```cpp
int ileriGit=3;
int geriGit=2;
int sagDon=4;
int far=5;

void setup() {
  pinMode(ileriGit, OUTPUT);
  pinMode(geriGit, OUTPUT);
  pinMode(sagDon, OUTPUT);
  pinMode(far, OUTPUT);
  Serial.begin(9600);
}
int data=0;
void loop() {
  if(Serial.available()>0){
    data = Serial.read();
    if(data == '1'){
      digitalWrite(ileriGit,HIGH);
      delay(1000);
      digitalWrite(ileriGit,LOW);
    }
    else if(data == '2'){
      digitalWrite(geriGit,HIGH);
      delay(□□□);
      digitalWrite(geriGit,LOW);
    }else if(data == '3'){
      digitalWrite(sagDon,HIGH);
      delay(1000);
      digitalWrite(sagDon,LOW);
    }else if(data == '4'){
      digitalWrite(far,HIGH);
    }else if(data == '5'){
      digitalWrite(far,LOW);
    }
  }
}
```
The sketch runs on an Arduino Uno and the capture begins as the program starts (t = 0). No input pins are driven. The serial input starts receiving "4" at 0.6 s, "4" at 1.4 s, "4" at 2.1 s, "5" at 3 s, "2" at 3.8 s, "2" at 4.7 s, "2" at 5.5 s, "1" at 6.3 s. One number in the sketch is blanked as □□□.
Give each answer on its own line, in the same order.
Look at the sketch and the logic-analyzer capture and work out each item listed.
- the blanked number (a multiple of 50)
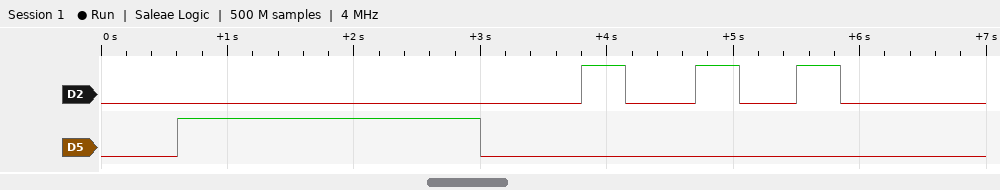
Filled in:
350
